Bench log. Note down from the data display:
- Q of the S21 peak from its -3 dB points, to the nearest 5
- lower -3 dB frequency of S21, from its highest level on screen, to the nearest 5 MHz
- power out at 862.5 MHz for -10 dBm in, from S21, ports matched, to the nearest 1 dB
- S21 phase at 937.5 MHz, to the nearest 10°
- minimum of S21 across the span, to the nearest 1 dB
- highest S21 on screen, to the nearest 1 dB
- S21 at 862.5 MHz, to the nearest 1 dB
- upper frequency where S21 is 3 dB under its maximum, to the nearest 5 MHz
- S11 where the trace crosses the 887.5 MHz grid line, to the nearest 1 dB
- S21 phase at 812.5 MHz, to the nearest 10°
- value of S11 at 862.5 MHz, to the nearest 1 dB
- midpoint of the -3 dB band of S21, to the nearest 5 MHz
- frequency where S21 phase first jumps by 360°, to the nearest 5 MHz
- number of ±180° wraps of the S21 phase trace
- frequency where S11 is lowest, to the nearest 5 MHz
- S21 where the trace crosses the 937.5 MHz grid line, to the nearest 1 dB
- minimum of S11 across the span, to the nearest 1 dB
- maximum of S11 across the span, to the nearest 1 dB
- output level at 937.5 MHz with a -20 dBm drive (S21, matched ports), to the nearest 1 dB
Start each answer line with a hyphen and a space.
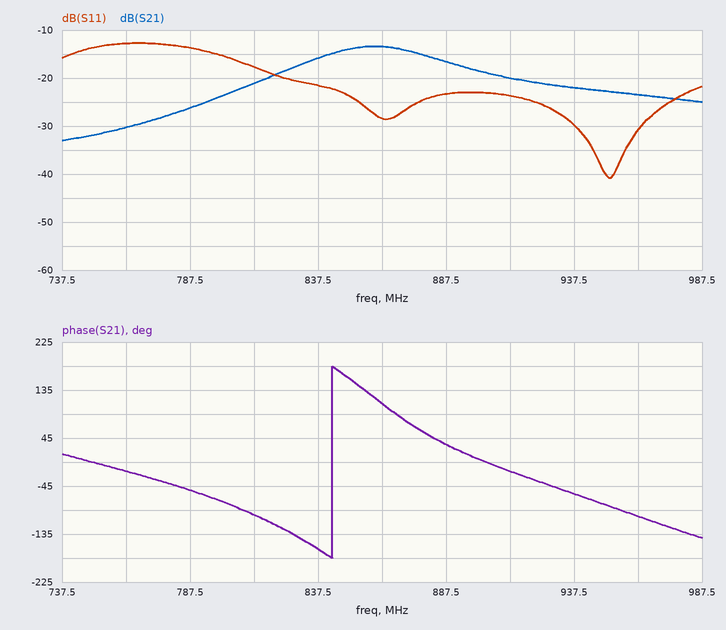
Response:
- 15
- 835 MHz
- -23 dBm
- -60°
- -33 dB
- -13 dB
- -13 dB
- 885 MHz
- -23 dB
- -100°
- -28 dB
- 860 MHz
- 845 MHz
- 1
- 950 MHz
- -22 dB
- -41 dB
- -13 dB
- -42 dBm
